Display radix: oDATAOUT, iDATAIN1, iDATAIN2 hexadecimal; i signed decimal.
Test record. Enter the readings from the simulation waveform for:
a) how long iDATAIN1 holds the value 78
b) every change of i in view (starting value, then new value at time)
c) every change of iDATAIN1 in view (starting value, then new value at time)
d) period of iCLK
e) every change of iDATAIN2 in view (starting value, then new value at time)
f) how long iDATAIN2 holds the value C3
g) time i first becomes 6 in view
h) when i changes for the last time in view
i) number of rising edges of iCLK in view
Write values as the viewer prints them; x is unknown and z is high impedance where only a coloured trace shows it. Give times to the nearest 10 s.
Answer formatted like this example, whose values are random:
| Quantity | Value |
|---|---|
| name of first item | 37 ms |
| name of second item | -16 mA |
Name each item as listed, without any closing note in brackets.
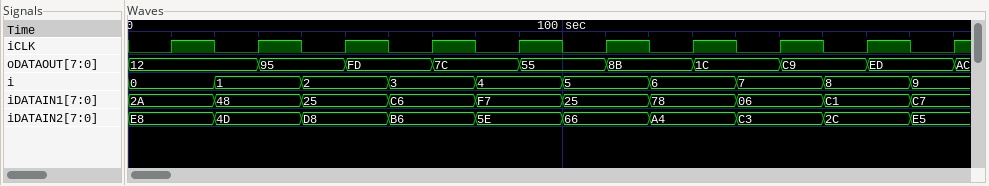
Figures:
| Quantity | Value |
|---|---|
| how long iDATAIN1 holds the value 78 | 20 s |
| every change of i in view | 0, 1 at 20 s, 2 at 40 s, 3 at 60 s, 4 at 80 s, 5 at 100 s, 6 at 120 s, 7 at 140 s, 8 at 160 s, 9 at 180 s |
| every change of iDATAIN1 in view | 2A, 48 at 20 s, 25 at 40 s, C6 at 60 s, F7 at 80 s, 25 at 100 s, 78 at 120 s, 06 at 140 s, C1 at 160 s, C7 at 180 s |
| period of iCLK | 20 s |
| every change of iDATAIN2 in view | E8, 4D at 20 s, D8 at 40 s, B6 at 60 s, 5E at 80 s, 66 at 100 s, A4 at 120 s, C3 at 140 s, 2C at 160 s, E5 at 180 s |
| how long iDATAIN2 holds the value C3 | 20 s |
| time i first becomes 6 in view | 120 s |
| when i changes for the last time in view | 180 s |
| number of rising edges of iCLK in view | 10 |
